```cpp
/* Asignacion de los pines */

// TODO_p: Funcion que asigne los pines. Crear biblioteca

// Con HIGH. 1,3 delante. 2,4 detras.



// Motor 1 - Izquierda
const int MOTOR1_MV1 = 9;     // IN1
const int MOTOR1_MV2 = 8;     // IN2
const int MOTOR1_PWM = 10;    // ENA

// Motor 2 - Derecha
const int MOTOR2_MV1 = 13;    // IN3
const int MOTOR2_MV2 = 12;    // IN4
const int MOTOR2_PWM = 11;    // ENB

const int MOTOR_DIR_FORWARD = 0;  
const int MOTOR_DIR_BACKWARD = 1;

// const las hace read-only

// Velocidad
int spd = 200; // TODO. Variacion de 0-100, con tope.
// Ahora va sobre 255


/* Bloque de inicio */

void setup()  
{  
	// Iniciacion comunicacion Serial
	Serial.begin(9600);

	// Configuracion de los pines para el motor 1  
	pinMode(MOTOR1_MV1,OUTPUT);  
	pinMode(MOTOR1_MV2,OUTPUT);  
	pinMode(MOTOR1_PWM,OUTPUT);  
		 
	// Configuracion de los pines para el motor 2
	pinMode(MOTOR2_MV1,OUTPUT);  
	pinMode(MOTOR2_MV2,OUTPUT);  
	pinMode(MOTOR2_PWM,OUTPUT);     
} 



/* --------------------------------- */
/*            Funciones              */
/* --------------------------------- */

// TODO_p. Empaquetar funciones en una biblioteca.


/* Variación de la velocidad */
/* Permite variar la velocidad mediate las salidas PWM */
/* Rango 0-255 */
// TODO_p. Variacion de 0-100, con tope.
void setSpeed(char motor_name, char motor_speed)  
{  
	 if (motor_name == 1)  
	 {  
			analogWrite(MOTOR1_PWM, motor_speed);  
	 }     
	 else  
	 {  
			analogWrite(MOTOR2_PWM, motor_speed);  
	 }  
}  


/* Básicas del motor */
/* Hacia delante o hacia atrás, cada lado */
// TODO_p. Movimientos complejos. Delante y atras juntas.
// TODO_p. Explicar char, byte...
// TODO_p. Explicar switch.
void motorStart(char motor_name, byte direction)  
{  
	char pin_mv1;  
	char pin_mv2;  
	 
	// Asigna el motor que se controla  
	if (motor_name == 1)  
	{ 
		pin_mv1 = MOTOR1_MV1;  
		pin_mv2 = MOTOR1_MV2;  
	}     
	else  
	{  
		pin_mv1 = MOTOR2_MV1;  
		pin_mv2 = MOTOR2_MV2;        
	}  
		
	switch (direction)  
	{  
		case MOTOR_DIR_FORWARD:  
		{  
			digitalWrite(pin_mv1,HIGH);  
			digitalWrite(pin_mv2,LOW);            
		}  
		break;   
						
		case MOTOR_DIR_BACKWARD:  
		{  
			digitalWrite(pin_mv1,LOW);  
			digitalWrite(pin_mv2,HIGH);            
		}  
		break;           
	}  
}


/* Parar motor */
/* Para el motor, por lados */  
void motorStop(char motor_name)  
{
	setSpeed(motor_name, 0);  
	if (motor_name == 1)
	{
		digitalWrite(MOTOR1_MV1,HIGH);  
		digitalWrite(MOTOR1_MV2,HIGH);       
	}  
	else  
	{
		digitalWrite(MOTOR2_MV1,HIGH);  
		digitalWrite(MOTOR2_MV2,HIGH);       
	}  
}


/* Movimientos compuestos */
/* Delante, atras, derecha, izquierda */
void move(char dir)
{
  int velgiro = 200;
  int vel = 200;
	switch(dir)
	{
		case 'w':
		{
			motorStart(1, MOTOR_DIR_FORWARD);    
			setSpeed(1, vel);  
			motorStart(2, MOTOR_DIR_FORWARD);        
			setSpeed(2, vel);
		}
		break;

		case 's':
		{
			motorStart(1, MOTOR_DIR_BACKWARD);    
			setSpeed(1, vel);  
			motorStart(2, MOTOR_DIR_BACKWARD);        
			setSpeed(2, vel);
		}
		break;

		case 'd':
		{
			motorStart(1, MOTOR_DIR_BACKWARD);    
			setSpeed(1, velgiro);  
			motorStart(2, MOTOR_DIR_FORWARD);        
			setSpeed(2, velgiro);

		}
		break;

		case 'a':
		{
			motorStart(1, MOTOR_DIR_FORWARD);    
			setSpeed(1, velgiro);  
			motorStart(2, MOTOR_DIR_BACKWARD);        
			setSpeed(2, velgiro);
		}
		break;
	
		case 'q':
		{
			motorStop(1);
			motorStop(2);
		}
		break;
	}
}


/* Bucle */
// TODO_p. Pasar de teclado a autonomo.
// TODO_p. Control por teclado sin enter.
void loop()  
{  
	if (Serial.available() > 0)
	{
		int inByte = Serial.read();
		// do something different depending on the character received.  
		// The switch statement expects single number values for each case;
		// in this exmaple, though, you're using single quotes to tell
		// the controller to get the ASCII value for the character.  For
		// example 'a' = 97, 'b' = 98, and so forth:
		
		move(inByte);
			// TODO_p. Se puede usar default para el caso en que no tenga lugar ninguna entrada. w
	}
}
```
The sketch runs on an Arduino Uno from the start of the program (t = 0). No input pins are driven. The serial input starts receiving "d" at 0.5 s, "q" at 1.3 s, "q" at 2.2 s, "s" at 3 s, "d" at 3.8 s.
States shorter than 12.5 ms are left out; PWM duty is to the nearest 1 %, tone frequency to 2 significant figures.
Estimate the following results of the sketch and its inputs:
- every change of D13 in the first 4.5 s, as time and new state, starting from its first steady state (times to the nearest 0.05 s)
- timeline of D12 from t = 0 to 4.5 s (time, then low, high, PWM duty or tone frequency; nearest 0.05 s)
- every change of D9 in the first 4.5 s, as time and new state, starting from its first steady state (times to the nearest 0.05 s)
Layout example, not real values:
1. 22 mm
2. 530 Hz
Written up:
1. 0 s low; 0.5 s high; 3 s low; 3.8 s high
2. 0 s low; 1.3 s high; 3.8 s low
3. 0 s low; 1.3 s high; 3 s low
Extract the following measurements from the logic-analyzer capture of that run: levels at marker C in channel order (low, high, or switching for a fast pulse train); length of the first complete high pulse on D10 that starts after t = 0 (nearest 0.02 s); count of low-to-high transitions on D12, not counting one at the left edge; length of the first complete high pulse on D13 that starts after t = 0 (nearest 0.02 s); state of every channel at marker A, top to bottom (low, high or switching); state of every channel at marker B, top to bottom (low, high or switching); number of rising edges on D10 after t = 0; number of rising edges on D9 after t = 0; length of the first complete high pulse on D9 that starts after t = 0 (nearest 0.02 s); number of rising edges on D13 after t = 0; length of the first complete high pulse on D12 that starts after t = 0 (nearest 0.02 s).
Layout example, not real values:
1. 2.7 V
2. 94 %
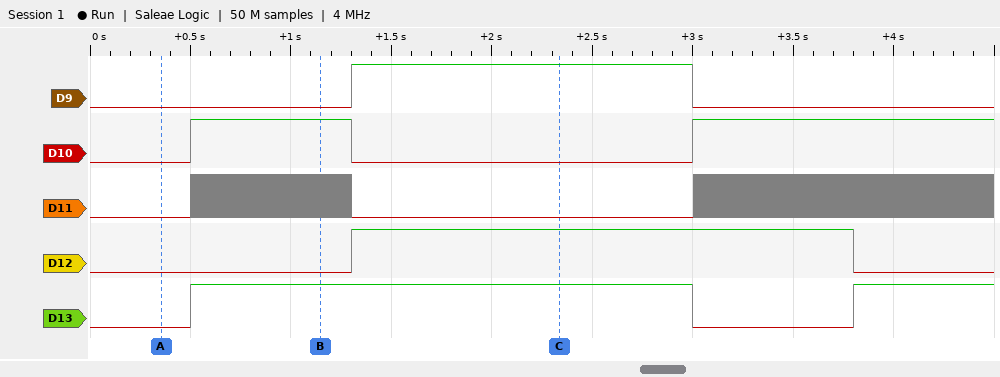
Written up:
1. D9 high, D10 low, D11 low, D12 high, D13 high
2. 0.80 s
3. 1
4. 2.50 s
5. D9 low, D10 low, D11 low, D12 low, D13 low
6. D9 low, D10 high, D11 switching, D12 low, D13 high
7. 2
8. 1
9. 1.70 s
10. 2
11. 2.50 s
